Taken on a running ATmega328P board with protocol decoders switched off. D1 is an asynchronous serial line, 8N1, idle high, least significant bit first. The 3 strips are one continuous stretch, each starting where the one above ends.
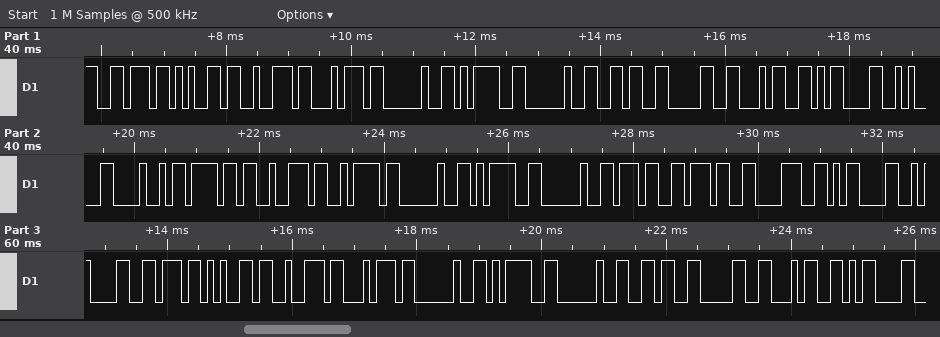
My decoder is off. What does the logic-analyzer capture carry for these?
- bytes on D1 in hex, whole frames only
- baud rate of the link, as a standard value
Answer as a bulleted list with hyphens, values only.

- 76 65 72 74 20 3D 20 36 30 34 0D 0A 48 6F 72 7A 20 3D 20 37 37 38 0D 0A 76 65 72 74 20 3D 20 36 30 34 0D
- 9600 baud
